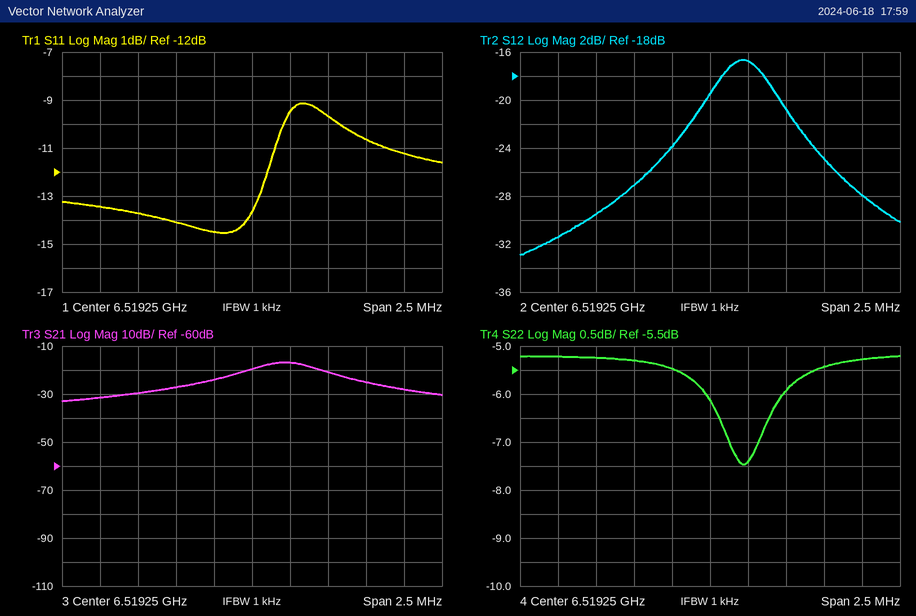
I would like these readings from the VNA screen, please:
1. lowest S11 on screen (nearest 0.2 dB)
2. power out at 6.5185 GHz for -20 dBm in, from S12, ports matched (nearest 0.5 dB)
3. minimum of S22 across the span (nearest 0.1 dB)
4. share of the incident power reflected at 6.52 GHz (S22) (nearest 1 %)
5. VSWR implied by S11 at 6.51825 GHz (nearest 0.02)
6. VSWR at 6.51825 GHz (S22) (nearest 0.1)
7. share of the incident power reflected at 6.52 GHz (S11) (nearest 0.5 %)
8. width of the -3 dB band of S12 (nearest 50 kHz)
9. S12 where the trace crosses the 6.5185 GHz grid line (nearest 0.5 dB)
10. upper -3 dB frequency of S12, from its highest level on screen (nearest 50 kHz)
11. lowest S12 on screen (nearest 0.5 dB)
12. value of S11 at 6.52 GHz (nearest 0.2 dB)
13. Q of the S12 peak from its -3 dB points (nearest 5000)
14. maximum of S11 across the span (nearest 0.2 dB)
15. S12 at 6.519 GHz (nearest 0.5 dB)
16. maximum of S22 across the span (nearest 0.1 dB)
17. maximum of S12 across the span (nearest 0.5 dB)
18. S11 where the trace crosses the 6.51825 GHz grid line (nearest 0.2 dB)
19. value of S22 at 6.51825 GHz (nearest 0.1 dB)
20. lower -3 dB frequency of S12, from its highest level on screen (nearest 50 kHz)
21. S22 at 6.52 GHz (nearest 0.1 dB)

-14.6 dB
-49.5 dBm
-7.5 dB
29 %
1.54
3.4
8.5 %
450 kHz
-29.5 dB
6.51970 GHz
-33.0 dB
-10.6 dB
15000
-9.2 dB
-24.0 dB
-5.2 dB
-16.5 dB
-13.4 dB
-5.2 dB
6.51925 GHz
-5.4 dB
